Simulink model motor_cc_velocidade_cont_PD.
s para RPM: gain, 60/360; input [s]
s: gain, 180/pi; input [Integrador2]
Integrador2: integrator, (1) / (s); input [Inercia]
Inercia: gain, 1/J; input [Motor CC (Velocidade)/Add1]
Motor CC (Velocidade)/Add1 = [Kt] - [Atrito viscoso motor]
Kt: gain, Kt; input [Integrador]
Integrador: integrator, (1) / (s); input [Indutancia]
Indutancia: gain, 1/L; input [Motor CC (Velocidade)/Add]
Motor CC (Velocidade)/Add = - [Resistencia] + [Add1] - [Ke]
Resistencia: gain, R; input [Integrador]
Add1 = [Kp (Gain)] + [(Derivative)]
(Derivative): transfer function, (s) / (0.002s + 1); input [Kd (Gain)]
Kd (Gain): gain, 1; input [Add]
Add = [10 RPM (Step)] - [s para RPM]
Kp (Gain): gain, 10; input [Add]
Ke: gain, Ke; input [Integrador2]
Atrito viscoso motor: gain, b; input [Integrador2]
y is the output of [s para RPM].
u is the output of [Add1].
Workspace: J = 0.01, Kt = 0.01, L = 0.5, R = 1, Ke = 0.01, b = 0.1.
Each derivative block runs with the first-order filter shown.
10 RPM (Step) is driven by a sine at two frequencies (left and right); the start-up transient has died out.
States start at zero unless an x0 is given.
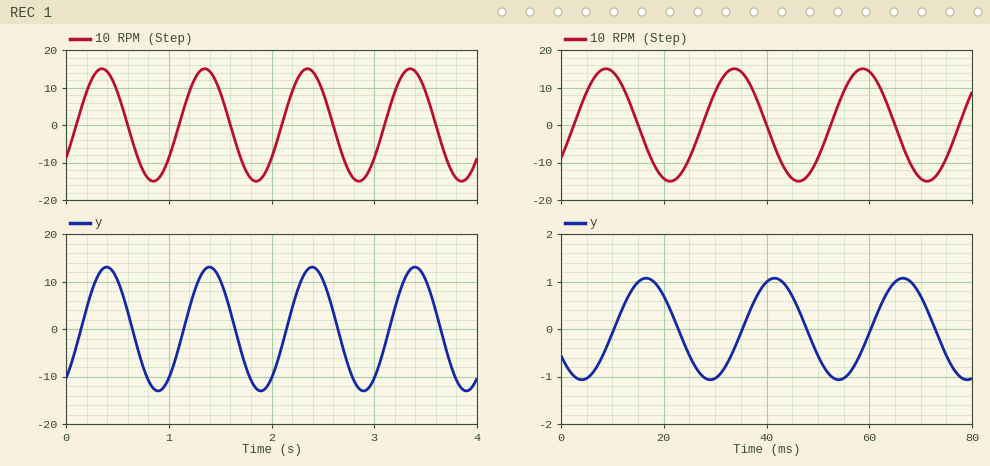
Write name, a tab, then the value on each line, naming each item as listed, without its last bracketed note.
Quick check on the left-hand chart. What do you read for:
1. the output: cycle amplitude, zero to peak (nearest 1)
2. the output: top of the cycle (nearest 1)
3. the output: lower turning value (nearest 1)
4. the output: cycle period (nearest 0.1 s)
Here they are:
the output: cycle amplitude, zero to peak	13
the output: top of the cycle	13
the output: lower turning value	-13
the output: cycle period	1.0 s
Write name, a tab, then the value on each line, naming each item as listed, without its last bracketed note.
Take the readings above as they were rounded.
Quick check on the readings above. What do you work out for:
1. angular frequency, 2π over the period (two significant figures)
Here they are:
angular frequency, 2π over the period	6.3 rad/s
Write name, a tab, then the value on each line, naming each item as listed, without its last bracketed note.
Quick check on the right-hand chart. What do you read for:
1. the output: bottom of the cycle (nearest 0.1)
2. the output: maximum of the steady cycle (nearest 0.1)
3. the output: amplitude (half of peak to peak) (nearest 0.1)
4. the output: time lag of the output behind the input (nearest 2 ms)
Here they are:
the output: bottom of the cycle	-1.1
the output: maximum of the steady cycle	1.1
the output: amplitude (half of peak to peak)	1.1
the output: time lag of the output behind the input	8 ms
